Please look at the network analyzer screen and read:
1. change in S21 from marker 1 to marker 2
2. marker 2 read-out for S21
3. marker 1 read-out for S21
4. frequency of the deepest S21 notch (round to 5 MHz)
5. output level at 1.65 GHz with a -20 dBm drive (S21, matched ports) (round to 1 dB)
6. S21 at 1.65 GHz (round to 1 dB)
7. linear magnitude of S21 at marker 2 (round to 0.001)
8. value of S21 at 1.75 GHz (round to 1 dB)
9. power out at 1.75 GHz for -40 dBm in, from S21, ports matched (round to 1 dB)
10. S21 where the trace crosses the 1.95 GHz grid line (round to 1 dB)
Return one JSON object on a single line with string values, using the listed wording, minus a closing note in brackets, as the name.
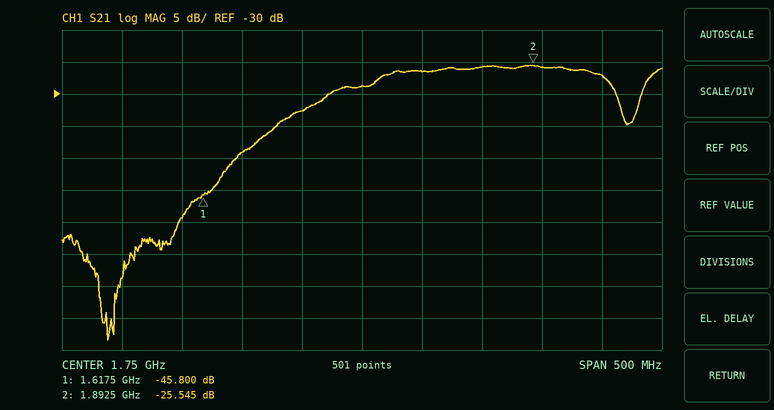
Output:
{"change in S21 from marker 1 to marker 2": "20.255 dB", "marker 2 read-out for S21": "-25.545 dB", "marker 1 read-out for S21": "-45.800 dB", "frequency of the deepest S21 notch": "1.540 GHz", "output level at 1.65 GHz with a -20 dBm drive (S21, matched ports)": "-59 dBm", "S21 at 1.65 GHz": "-39 dB", "linear magnitude of S21 at marker 2": "0.053", "value of S21 at 1.75 GHz": "-29 dB", "power out at 1.75 GHz for -40 dBm in, from S21, ports matched": "-69 dBm", "S21 where the trace crosses the 1.95 GHz grid line": "-27 dB"}
